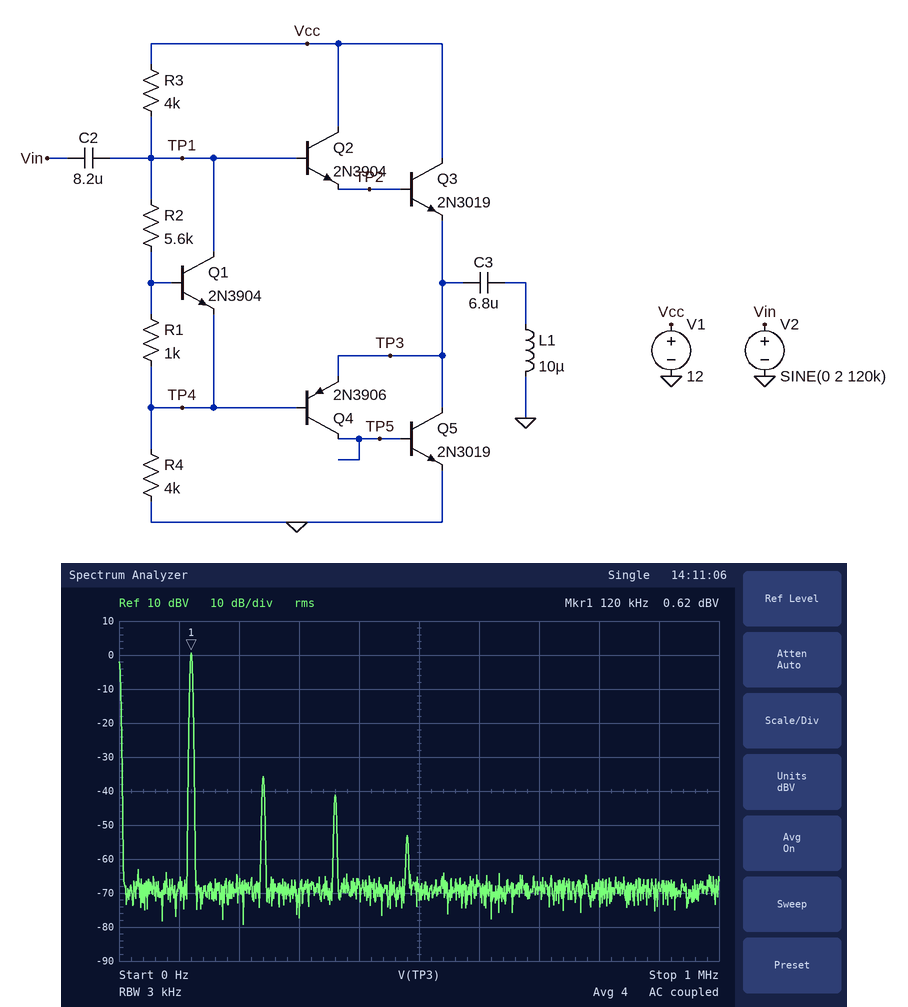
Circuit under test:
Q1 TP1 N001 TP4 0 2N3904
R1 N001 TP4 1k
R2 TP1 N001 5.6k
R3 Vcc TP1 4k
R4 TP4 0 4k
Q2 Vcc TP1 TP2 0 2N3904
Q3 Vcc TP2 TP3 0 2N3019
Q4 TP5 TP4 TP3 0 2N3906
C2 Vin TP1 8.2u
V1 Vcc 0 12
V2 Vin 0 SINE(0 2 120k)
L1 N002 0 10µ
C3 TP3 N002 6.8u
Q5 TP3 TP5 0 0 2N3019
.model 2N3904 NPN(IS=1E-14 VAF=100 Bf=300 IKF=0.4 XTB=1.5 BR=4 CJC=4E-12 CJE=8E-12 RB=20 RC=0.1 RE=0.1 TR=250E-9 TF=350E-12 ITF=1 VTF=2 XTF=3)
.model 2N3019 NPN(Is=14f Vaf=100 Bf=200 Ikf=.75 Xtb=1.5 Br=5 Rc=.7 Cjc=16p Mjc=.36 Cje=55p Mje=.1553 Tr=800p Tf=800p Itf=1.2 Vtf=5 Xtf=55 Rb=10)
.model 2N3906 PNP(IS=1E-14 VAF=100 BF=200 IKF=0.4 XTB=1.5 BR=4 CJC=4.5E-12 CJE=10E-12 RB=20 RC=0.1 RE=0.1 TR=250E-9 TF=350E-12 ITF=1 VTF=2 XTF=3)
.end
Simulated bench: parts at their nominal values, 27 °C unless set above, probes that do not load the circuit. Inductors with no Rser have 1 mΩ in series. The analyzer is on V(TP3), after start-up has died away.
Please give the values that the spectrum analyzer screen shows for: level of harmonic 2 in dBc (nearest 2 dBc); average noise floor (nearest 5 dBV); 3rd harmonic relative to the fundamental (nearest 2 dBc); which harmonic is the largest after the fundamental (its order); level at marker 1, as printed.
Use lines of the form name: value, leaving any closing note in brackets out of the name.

level of harmonic 2 in dBc: -36 dBc
average noise floor: -70 dBV
3rd harmonic relative to the fundamental: -42 dBc
which harmonic is the largest after the fundamental: 2
level at marker 1, as printed: 0.62 dBV
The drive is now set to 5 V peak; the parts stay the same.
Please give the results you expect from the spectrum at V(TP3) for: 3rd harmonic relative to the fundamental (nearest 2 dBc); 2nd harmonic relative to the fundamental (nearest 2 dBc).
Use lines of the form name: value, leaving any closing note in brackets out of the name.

3rd harmonic relative to the fundamental: -30 dBc
2nd harmonic relative to the fundamental: -32 dBc
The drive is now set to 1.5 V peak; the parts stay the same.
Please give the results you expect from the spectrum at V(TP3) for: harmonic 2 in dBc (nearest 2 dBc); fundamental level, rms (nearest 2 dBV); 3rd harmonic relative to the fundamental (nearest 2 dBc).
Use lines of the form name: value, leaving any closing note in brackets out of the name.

harmonic 2 in dBc: -38 dBc
fundamental level, rms: -2 dBV
3rd harmonic relative to the fundamental: -46 dBc
